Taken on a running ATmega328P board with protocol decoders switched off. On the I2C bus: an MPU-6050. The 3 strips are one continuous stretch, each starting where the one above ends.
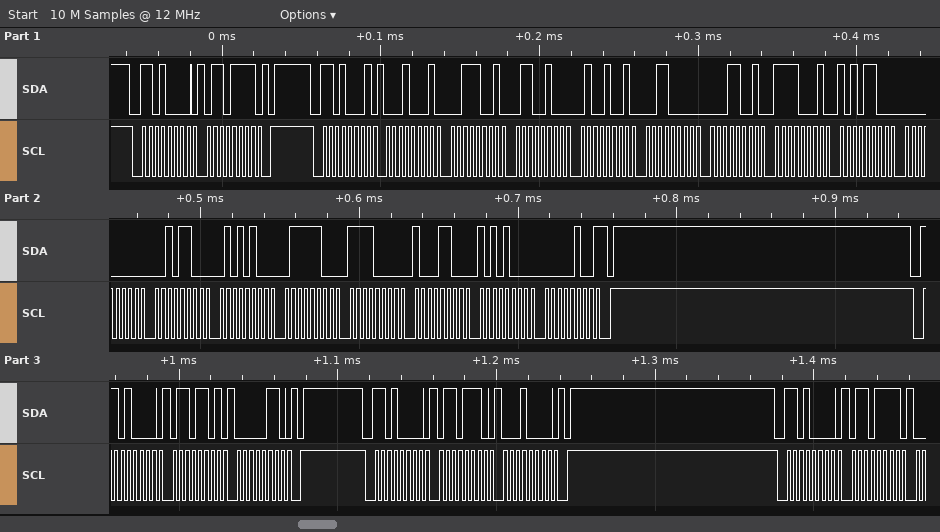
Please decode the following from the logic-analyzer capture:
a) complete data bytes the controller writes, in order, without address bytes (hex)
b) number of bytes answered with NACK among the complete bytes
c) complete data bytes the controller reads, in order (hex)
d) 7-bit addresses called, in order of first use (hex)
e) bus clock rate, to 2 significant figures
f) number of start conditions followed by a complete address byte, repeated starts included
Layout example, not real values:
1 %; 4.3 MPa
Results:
6F 6D 06 6E 10 6F; 1; 11 39 64 49 30 19 F1 AC 00 2C 54 7C F0 8C A8 04; 0x68; 250 kHz; 5
